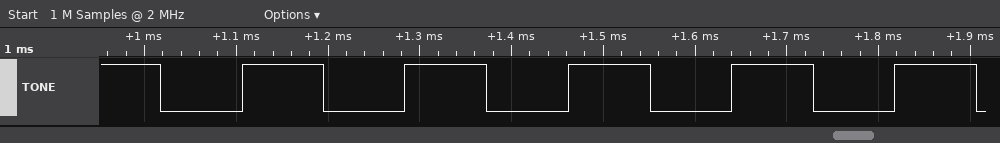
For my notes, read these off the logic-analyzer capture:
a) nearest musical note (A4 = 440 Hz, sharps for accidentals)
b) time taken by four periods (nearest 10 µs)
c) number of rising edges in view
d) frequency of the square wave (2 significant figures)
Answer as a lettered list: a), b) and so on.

a) F8
b) 720 µs
c) 5
d) 5.6 kHz
